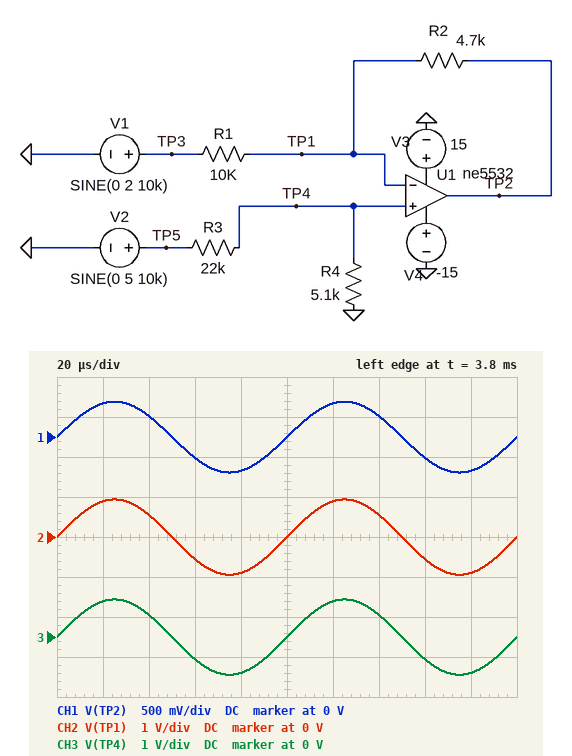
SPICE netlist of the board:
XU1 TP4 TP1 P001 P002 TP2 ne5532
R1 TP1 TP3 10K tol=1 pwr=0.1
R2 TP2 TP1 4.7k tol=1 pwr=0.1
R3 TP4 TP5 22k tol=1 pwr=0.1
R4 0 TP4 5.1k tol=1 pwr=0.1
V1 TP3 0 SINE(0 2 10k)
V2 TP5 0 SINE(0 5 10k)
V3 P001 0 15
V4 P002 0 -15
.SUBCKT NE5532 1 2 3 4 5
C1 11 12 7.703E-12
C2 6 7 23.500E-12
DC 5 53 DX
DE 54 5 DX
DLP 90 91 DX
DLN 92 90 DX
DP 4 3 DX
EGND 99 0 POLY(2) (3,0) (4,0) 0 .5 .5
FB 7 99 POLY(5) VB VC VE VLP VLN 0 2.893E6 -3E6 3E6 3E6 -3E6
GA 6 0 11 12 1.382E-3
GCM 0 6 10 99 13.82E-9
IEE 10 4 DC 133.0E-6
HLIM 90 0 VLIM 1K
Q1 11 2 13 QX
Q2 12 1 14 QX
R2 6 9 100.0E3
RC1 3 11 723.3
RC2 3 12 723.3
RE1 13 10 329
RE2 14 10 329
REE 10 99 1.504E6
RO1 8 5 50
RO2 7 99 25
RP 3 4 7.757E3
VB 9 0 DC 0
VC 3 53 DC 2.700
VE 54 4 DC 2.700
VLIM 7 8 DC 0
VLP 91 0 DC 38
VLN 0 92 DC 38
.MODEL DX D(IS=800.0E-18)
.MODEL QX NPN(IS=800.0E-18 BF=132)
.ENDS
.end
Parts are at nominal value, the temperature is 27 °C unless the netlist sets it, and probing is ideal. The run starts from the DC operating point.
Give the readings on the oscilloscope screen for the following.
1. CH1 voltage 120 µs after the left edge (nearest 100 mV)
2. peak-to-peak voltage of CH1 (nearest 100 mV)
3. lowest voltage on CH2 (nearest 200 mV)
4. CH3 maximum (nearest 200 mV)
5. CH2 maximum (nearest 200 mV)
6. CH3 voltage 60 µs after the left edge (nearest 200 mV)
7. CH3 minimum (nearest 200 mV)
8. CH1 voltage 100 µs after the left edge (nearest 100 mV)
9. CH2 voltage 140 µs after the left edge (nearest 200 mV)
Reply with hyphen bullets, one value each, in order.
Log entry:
- 400 mV
- 900 mV
- -1.0 V
- 1.0 V
- 1.0 V
- -600 mV
- -1.0 V
- 0 V
- 600 mV
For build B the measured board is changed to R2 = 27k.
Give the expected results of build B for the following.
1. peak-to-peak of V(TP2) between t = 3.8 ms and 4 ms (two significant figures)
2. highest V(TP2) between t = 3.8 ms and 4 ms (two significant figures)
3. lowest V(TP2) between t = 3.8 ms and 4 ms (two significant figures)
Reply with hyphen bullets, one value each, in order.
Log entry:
- 3.8 V
- 1.9 V
- -1.9 V
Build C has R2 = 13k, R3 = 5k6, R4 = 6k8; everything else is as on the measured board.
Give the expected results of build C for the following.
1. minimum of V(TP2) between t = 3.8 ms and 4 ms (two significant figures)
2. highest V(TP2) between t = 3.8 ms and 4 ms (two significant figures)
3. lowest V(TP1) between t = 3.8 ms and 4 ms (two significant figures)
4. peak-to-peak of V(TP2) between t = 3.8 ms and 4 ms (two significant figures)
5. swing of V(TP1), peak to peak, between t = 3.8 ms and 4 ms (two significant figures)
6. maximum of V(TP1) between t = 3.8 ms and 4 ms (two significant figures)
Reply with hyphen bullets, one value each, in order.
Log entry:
- -3.7 V
- 3.7 V
- -2.7 V
- 7.4 V
- 5.5 V
- 2.7 V
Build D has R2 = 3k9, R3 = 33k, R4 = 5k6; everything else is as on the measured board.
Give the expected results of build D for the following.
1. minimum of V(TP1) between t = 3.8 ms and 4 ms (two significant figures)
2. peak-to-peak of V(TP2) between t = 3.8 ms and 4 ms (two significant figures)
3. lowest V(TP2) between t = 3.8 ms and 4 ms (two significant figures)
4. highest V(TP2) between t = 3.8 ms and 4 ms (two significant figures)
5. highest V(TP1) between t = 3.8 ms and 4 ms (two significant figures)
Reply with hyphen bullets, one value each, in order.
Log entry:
- -730 mV
- 460 mV
- -230 mV
- 230 mV
- 720 mV
